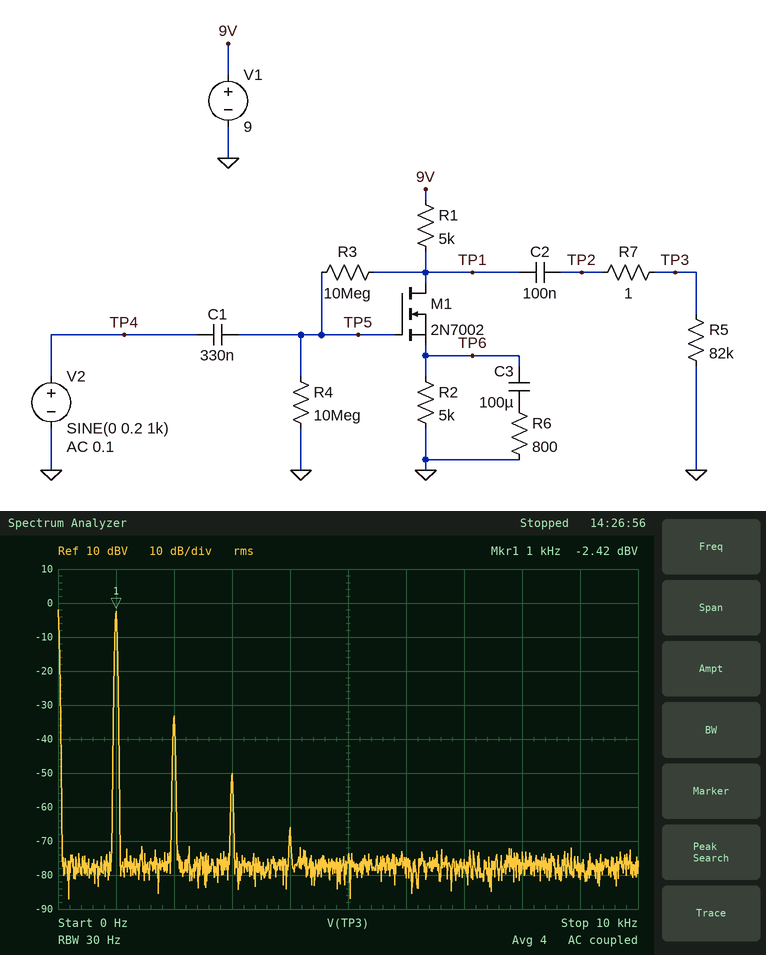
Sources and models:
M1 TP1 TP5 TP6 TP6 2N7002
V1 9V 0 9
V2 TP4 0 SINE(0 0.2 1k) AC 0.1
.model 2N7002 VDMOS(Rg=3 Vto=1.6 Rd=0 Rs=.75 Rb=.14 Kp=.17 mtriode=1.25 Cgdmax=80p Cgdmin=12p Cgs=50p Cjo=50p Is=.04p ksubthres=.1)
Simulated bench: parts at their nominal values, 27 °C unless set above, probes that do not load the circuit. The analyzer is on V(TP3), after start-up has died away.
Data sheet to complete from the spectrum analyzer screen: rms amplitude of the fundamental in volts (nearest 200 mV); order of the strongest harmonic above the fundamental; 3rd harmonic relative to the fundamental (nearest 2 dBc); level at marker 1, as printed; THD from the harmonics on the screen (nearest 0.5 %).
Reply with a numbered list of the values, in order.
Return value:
1. 800 mV
2. 2
3. -48 dBc
4. -2.42 dBV
5. 3.0 %
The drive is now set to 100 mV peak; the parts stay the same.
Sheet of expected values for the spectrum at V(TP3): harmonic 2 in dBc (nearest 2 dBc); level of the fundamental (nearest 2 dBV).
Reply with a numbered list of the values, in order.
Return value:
1. -38 dBc
2. -8 dBV
